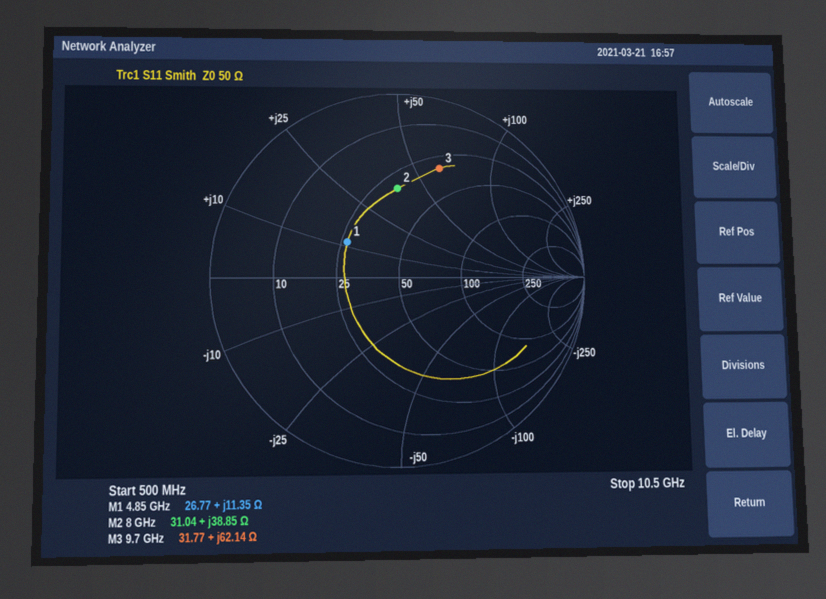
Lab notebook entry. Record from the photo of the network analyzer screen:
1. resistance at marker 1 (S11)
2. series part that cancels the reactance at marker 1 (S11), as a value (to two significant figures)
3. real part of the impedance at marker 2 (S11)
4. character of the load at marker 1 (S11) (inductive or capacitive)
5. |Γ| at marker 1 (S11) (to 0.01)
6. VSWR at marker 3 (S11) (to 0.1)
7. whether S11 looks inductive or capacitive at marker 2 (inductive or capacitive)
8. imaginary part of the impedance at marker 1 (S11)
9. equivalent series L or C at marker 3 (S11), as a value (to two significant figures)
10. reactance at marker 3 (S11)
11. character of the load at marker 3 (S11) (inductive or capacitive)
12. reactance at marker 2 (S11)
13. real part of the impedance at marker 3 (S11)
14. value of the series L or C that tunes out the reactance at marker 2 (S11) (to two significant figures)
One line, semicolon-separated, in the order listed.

26.77 Ω; 2.9 pF; 31.04 Ω; inductive; 0.33; 4.4; inductive; +11.35 Ω; 1.0 nH; +62.14 Ω; inductive; +38.85 Ω; 31.77 Ω; 510 fF
